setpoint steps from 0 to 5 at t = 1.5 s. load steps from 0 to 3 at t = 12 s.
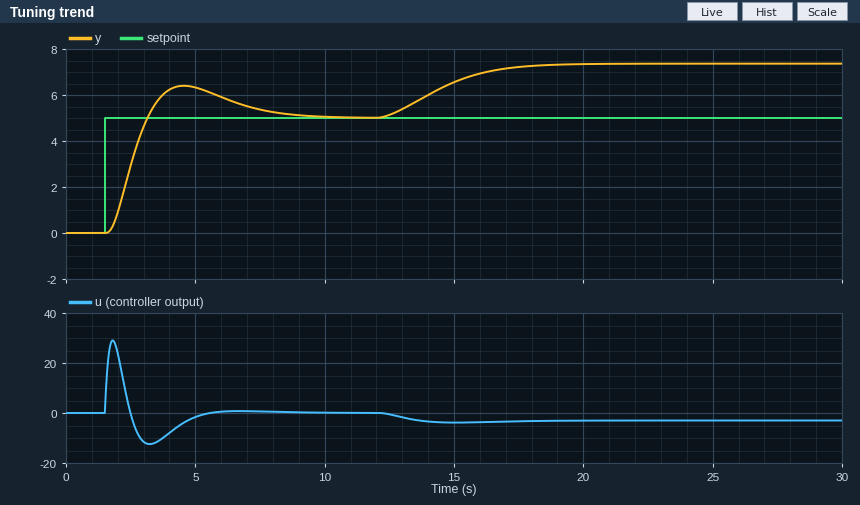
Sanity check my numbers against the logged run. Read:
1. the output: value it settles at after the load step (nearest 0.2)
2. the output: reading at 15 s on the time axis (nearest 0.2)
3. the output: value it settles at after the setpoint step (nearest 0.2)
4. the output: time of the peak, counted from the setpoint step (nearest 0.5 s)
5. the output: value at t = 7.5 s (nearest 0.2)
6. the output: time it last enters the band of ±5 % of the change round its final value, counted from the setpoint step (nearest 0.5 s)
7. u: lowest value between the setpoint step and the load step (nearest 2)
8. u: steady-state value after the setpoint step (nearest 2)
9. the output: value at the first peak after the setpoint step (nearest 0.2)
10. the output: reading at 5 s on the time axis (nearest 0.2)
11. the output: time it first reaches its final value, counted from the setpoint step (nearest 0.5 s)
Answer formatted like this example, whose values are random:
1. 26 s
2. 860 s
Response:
1. 7.4
2. 6.6
3. 5.0
4. 3.0 s
5. 5.4
6. 6.5 s
7. -12
8. 0
9. 6.4
10. 6.4
11. 1.5 s
